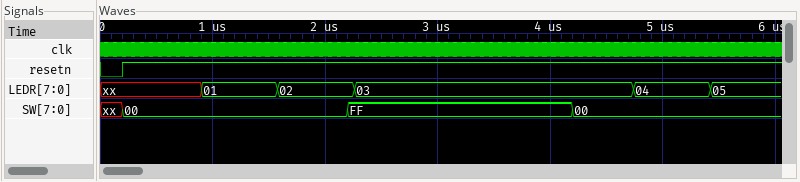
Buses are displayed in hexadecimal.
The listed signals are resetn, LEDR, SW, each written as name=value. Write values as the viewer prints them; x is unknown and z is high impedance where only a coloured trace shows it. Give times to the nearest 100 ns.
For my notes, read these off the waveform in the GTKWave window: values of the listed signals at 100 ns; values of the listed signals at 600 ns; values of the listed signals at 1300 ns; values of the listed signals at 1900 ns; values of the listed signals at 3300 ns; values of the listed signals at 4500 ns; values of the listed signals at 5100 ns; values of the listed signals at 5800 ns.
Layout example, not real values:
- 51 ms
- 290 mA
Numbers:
- resetn=0, LEDR=xx, SW=xx
- resetn=1, LEDR=xx, SW=00
- resetn=1, LEDR=01, SW=00
- resetn=1, LEDR=02, SW=00
- resetn=1, LEDR=03, SW=FF
- resetn=1, LEDR=03, SW=00
- resetn=1, LEDR=04, SW=00
- resetn=1, LEDR=05, SW=00
